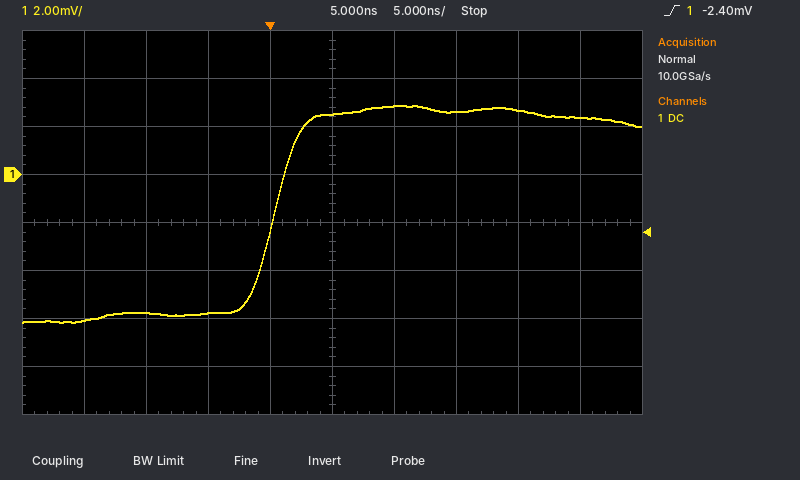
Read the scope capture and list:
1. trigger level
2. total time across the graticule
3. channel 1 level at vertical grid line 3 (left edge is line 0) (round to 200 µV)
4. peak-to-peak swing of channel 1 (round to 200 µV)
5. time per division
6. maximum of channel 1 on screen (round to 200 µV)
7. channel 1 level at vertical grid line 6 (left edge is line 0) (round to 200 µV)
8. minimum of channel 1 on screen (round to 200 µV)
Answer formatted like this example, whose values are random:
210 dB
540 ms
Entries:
-2.40 mV
50 ns
-5.8 mV
9.0 mV
5 ns
2.8 mV
2.8 mV
-6.2 mV
